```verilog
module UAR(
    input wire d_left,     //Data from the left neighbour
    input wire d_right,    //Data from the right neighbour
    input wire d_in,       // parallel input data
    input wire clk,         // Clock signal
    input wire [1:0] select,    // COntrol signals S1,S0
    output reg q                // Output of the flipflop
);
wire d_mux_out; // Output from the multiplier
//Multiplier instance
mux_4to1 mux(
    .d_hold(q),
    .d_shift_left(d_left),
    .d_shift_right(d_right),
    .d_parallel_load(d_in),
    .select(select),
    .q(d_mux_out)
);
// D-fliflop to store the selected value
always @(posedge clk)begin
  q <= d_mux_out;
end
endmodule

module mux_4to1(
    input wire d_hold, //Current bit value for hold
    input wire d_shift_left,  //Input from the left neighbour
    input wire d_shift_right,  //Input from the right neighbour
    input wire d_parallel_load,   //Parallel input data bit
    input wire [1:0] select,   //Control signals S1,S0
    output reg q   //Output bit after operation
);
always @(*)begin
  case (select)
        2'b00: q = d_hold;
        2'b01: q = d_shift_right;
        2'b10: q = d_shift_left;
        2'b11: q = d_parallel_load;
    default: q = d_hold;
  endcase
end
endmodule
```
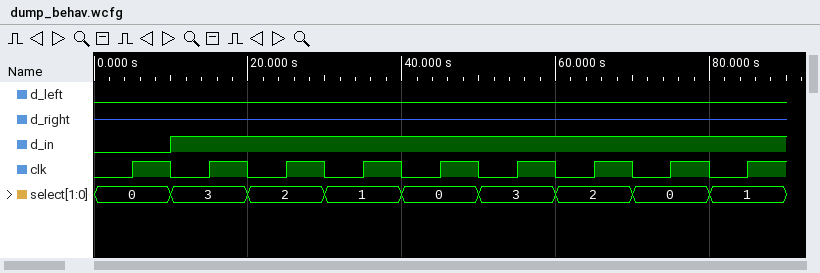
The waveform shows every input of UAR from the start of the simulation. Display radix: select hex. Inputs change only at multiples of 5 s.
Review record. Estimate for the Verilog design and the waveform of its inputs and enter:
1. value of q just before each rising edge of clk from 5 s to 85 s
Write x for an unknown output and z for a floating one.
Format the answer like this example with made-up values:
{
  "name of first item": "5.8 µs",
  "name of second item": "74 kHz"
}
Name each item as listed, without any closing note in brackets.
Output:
{
  "value of q just before each rising edge of clk from 5 s to 85 s": "x x 1 0 z z 1 0 0"
}
